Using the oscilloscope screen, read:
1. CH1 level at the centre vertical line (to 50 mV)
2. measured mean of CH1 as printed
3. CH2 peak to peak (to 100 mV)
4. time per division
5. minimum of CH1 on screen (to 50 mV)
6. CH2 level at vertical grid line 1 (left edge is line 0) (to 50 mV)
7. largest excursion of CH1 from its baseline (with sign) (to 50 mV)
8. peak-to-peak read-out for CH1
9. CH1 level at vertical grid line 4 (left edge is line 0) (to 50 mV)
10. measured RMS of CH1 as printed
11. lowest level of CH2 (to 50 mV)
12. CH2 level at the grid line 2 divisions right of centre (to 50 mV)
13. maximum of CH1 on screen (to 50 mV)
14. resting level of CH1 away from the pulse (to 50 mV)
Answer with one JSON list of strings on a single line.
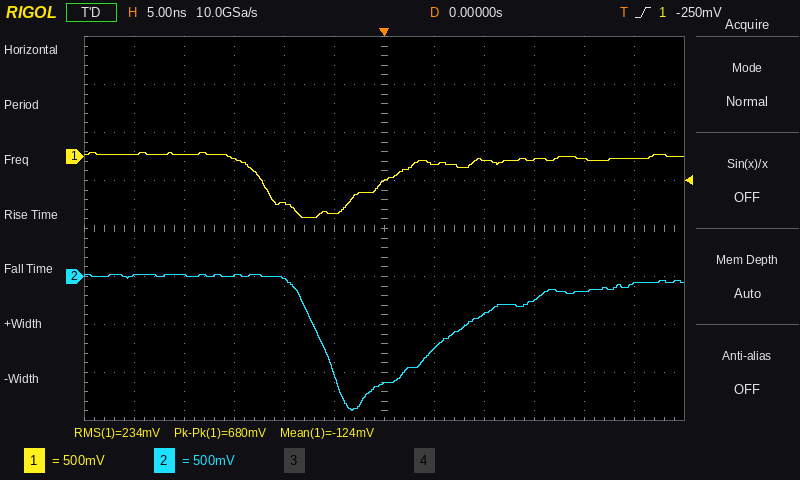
["-250 mV", "-124 mV", "1.40 V", "5 ns", "-650 mV", "0 mV", "-600 mV", "680 mV", "-500 mV", "234 mV", "-1.40 V", "-400 mV", "50 mV", "-50 mV"]
